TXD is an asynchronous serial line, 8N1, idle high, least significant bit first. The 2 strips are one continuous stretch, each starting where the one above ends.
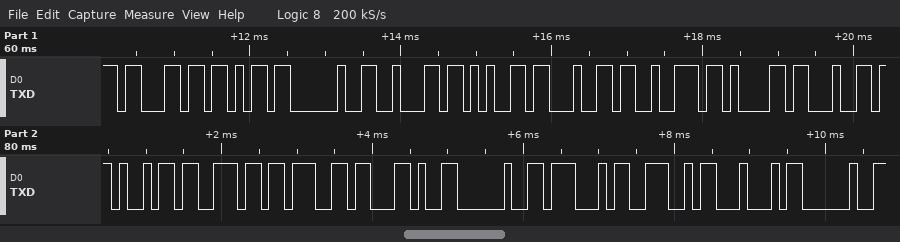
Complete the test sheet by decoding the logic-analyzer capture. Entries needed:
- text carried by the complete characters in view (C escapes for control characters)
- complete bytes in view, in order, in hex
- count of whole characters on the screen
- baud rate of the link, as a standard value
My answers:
"ck bedrading, GND "
63 6B 20 62 65 64 72 61 64 69 6E 67 2C 20 47 4E 44 20
18
9600 baud
